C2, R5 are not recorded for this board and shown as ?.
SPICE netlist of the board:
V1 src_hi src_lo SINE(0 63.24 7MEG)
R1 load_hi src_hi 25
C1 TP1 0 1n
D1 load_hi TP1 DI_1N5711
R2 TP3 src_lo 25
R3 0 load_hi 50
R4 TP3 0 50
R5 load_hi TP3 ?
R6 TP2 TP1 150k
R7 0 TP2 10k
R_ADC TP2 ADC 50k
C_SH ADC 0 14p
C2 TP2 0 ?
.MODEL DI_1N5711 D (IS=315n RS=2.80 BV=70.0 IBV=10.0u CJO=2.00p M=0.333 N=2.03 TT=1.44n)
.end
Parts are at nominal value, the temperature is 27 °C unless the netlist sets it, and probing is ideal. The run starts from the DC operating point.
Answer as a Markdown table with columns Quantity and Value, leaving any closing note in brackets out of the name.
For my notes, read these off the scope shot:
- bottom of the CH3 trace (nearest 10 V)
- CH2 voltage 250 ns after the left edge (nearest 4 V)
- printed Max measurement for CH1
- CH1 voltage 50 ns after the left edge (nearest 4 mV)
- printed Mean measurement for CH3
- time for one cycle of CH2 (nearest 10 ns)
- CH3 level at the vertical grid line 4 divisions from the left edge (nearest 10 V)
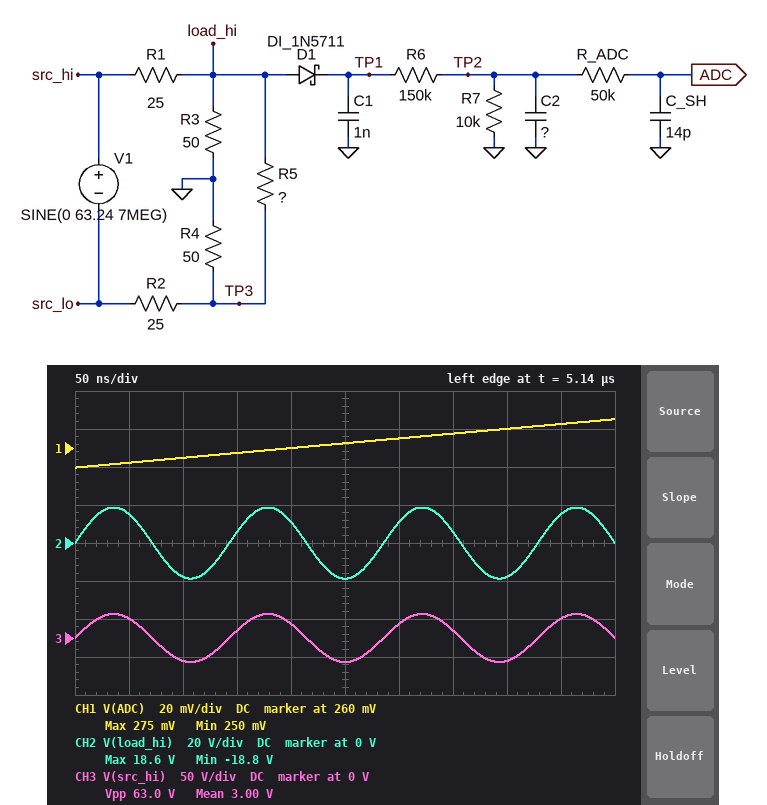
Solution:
| Quantity | Value |
|---|---|
| bottom of the CH3 trace | -30 V |
| CH2 voltage 250 ns after the left edge | -20 V |
| printed Max measurement for CH1 | 275 mV |
| CH1 voltage 50 ns after the left edge | 252 mV |
| printed Mean measurement for CH3 | 3.00 V |
| time for one cycle of CH2 | 140 ns |
| CH3 level at the vertical grid line 4 divisions from the left edge | 20 V |
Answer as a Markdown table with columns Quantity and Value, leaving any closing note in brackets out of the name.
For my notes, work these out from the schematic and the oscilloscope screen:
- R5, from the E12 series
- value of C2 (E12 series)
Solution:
| Quantity | Value |
|---|---|
| R5, from the E12 series | 270 Ω |
| value of C2 | 1.8 nF |
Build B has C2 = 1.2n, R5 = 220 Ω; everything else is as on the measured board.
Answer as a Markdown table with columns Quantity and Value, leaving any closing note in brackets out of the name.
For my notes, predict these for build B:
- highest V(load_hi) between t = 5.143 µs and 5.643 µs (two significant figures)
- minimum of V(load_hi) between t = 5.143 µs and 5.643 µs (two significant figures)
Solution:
| Quantity | Value |
|---|---|
| highest V(load_hi) between t = 5.143 µs and 5.643 µs | 18 V |
| minimum of V(load_hi) between t = 5.143 µs and 5.643 µs | -18 V |
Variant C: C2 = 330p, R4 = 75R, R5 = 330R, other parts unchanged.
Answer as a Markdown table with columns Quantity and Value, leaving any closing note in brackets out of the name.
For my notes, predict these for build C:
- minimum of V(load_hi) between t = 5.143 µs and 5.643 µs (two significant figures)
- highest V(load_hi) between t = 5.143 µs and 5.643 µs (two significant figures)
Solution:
| Quantity | Value |
|---|---|
| minimum of V(load_hi) between t = 5.143 µs and 5.643 µs | -16 V |
| highest V(load_hi) between t = 5.143 µs and 5.643 µs | 16 V |
